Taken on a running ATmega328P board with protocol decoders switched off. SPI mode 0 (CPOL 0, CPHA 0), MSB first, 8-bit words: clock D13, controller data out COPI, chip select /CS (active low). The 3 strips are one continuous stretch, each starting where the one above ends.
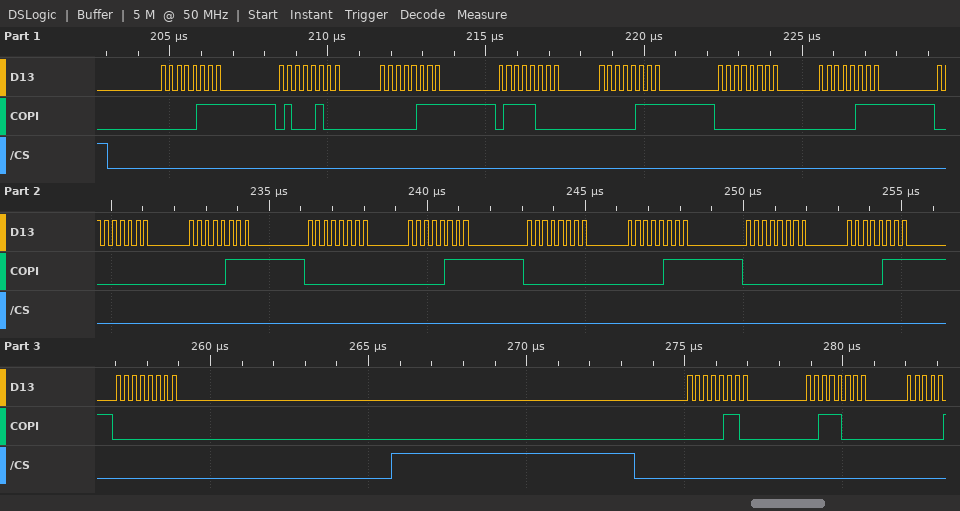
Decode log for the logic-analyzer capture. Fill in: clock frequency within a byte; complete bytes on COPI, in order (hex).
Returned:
4 MHz
07 44 07 78 07 00 07 00 07 00 07 00 07 00 07 00 06 38
